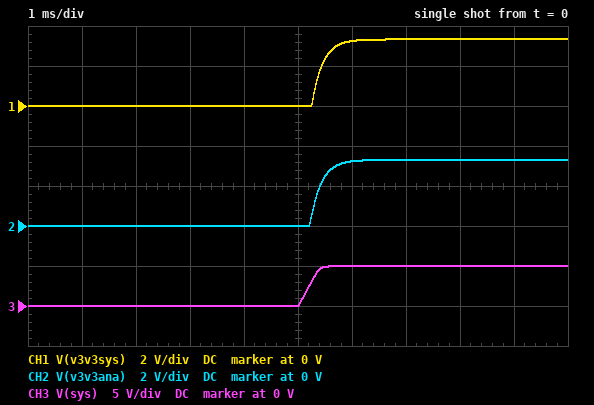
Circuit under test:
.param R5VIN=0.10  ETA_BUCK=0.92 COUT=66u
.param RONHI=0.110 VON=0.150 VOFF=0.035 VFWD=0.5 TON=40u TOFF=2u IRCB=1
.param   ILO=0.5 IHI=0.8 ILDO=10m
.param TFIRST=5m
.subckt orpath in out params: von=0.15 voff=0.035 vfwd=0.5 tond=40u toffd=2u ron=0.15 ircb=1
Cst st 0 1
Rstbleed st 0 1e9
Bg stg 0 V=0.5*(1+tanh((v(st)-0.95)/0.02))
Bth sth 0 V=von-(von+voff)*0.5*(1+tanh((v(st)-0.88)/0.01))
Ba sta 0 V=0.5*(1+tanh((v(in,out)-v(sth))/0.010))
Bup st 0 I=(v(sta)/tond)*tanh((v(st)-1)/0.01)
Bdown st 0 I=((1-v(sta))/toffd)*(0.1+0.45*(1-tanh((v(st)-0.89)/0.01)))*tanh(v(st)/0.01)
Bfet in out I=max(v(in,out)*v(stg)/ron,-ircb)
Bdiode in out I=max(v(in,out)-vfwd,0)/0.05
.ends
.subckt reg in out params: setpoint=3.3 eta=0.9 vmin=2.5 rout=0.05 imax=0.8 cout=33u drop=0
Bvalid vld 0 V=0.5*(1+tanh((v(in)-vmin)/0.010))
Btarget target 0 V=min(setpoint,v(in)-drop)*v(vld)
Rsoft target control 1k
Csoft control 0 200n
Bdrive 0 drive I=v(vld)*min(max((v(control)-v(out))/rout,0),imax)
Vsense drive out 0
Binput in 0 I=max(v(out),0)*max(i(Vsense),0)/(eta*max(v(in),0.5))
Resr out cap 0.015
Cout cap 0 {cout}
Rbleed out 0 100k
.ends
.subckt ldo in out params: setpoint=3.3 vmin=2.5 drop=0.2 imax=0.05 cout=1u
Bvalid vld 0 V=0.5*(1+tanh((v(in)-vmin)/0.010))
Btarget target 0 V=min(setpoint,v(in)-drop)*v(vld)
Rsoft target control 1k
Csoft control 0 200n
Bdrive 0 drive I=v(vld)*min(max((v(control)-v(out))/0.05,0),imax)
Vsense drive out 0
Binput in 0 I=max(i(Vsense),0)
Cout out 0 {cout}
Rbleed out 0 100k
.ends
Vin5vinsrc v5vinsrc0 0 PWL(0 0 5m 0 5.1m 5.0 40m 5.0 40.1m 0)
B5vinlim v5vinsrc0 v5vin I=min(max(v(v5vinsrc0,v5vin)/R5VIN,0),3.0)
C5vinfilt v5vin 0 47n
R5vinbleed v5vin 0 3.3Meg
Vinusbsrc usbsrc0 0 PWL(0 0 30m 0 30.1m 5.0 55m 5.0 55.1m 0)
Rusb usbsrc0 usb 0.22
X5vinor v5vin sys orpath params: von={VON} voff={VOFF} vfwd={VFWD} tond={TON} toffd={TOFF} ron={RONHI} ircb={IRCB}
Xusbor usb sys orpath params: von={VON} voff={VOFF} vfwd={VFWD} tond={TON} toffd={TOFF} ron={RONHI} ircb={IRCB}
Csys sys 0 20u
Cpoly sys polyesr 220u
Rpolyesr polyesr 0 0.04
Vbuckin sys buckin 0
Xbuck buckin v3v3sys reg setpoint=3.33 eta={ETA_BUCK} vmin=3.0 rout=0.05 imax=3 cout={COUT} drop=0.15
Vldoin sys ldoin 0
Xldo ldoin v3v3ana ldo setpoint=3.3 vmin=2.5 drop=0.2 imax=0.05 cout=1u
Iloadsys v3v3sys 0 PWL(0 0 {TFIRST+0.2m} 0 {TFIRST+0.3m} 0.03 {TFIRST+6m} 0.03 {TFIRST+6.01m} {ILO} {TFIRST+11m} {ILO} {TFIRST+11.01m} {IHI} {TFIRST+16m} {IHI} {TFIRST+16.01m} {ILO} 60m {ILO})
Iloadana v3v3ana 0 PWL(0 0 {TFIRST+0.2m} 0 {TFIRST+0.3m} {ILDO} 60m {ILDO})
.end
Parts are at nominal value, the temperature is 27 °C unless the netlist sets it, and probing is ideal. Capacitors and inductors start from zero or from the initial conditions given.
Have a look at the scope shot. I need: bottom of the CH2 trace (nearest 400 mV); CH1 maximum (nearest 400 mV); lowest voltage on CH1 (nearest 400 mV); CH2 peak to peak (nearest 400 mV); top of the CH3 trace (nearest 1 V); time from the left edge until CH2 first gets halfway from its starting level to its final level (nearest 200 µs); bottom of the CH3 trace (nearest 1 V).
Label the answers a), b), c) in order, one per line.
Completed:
a) 0 V
b) 3.2 V
c) 0 V
d) 3.2 V
e) 5 V
f) 5.4 ms
g) 0 V
